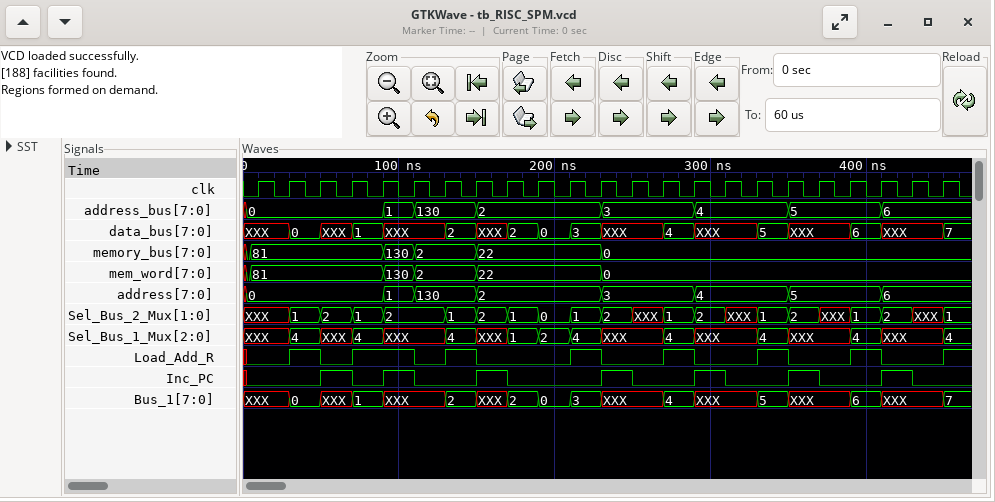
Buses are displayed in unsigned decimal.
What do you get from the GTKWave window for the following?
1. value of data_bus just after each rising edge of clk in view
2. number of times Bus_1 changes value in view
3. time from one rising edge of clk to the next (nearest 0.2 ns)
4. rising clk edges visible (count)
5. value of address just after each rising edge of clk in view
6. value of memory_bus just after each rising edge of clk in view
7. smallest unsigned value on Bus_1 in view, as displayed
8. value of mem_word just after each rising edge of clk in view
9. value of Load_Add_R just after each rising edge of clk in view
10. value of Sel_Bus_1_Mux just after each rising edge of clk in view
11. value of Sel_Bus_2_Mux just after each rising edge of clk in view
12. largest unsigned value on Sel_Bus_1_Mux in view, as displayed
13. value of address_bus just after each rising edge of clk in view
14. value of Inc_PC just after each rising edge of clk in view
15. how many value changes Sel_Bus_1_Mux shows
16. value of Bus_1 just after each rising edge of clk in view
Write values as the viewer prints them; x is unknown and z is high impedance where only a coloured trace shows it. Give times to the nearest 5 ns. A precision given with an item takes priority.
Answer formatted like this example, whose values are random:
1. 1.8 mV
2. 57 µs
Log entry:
1. XXX, 0, XXX, 1, XXX, XXX, 2, XXX, 2, 0, 3, XXX, XXX, 4, XXX, XXX, 5, XXX, XXX, 6, XXX, XXX, 7
2. 17
3. 20 ns
4. 23
5. 0, 0, 0, 0, 1, 130, 130, 2, 2, 2, 2, 3, 3, 3, 4, 4, 4, 5, 5, 5, 6, 6, 6
6. 81, 81, 81, 81, 130, 2, 2, 22, 22, 22, 22, 0, 0, 0, 0, 0, 0, 0, 0, 0, 0, 0, 0
7. 0
8. 81, 81, 81, 81, 130, 2, 2, 22, 22, 22, 22, 0, 0, 0, 0, 0, 0, 0, 0, 0, 0, 0, 0
9. 0 1 0 1 1 0 1 0 0 0 1 0 0 1 0 0 1 0 0 1 0 0 1
10. XXX, 4, XXX, 4, XXX, XXX, 4, XXX, 1, 2, 4, XXX, XXX, 4, XXX, XXX, 4, XXX, XXX, 4, XXX, XXX, 4
11. XXX, 1, 2, 1, 2, 2, 1, 2, 1, 0, 1, 2, XXX, 1, 2, XXX, 1, 2, XXX, 1, 2, XXX, 1
12. 4
13. 0, 0, 0, 0, 1, 130, 130, 2, 2, 2, 2, 3, 3, 3, 4, 4, 4, 5, 5, 5, 6, 6, 6
14. 0 0 1 0 1 0 0 1 0 0 0 1 0 0 1 0 0 1 0 0 1 0 0
15. 17
16. XXX, 0, XXX, 1, XXX, XXX, 2, XXX, 2, 0, 3, XXX, XXX, 4, XXX, XXX, 5, XXX, XXX, 6, XXX, XXX, 7
